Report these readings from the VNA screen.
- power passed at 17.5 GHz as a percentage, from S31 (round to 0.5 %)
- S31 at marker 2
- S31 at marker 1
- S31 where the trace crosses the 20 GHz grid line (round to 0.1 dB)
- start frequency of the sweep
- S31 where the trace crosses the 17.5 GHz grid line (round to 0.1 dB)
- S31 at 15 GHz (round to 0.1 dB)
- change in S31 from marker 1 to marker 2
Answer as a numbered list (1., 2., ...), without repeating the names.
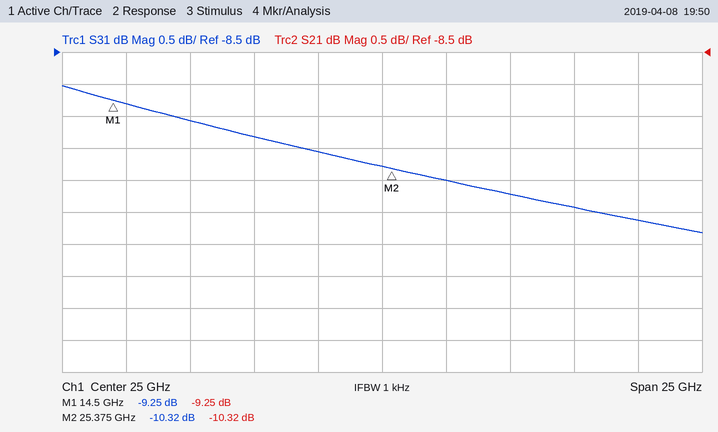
1. 11.0 %
2. -10.32 dB
3. -9.25 dB
4. -9.8 dB
5. 12.5 GHz
6. -9.6 dB
7. -9.3 dB
8. -1.07 dB
